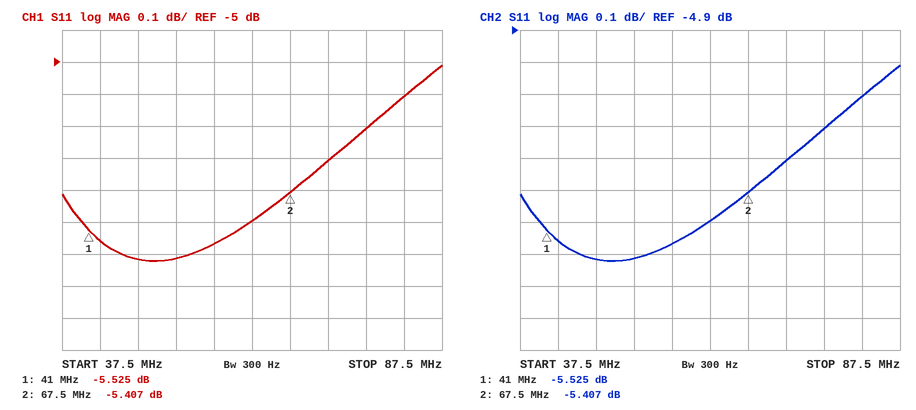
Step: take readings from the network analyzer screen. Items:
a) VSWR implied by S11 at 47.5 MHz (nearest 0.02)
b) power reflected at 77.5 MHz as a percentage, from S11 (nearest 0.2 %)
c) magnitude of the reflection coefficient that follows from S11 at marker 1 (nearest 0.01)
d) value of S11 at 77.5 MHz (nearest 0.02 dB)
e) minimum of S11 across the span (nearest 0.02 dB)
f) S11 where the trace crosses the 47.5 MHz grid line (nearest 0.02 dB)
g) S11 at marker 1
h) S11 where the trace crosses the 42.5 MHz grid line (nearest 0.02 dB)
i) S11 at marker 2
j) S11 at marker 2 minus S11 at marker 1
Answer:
3.20
30.2 %
0.53
-5.20 dB
-5.62 dB
-5.62 dB
-5.525 dB
-5.56 dB
-5.407 dB
0.118 dB
